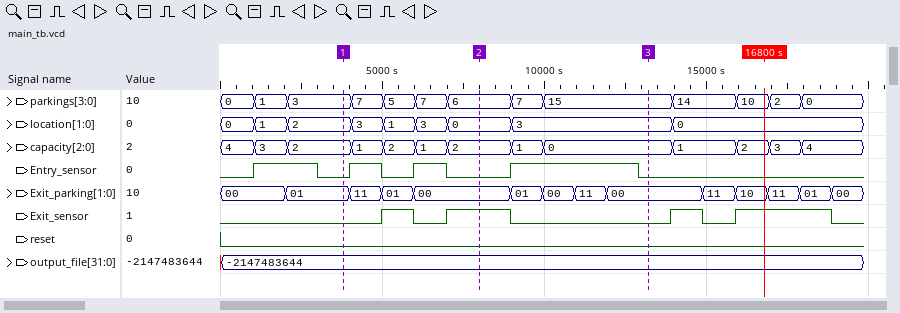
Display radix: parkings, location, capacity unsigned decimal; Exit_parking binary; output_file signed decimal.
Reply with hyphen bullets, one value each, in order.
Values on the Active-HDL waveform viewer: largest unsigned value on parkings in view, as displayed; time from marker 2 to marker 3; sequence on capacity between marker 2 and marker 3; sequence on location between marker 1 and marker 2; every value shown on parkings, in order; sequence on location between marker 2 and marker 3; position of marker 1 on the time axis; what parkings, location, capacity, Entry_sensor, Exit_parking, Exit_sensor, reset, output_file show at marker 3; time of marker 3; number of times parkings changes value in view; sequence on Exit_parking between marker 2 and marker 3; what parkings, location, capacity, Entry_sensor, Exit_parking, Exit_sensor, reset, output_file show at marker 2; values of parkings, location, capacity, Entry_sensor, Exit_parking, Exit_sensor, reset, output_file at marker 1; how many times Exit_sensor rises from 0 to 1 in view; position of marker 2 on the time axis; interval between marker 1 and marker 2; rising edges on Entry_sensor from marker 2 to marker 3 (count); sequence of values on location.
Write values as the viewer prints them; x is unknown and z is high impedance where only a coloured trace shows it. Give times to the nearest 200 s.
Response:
- 15
- 5200 s
- 2, 1, 0
- 2, 3, 1, 3, 0
- 0, 1, 3, 7, 5, 7, 6, 7, 15, 14, 10, 2, 0
- 0, 3
- 3800 s
- parkings=15, location=3, capacity=0, Entry_sensor=0, Exit_parking=00, Exit_sensor=0, reset=0, output_file=-2147483644
- 13200 s
- 12
- 00, 01, 00, 11, 00
- parkings=6, location=0, capacity=2, Entry_sensor=0, Exit_parking=00, Exit_sensor=1, reset=0, output_file=-2147483644
- parkings=3, location=2, capacity=2, Entry_sensor=0, Exit_parking=01, Exit_sensor=0, reset=0, output_file=-2147483644
- 4
- 8000 s
- 4200 s
- 1
- 0, 1, 2, 3, 1, 3, 0, 3, 0
